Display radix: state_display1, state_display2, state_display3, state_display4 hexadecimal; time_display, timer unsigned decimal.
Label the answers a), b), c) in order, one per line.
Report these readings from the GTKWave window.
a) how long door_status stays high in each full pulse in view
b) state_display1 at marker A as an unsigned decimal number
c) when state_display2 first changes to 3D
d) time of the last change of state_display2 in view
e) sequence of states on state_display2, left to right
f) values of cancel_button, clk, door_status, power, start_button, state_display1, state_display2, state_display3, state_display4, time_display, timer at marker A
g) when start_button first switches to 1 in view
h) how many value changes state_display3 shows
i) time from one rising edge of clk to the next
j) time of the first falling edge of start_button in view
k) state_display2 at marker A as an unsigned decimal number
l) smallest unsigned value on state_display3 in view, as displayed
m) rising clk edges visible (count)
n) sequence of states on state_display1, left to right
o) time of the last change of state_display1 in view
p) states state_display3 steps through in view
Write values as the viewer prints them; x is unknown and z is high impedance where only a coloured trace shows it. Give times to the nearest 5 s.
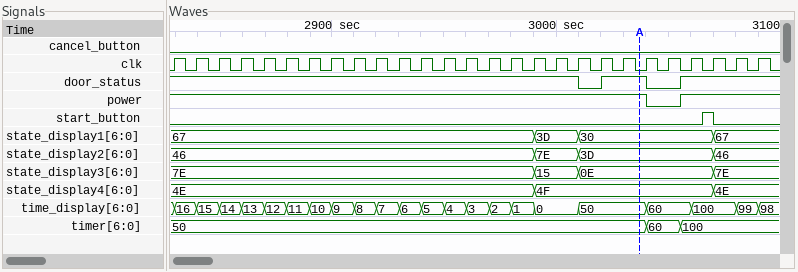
a) 20 s
b) 48
c) 3010 s
d) 3070 s
e) 46, 7E, 3D, 46
f) cancel_button=0, clk=0, door_status=1, power=1, start_button=0, state_display1=30, state_display2=3D, state_display3=0E, state_display4=4F, time_display=50, timer=50
g) 3065 s
h) 3
i) 10 s
j) 3070 s
k) 61
l) 0E
m) 27
n) 67, 3D, 30, 67
o) 3070 s
p) 7E, 15, 0E, 7E
